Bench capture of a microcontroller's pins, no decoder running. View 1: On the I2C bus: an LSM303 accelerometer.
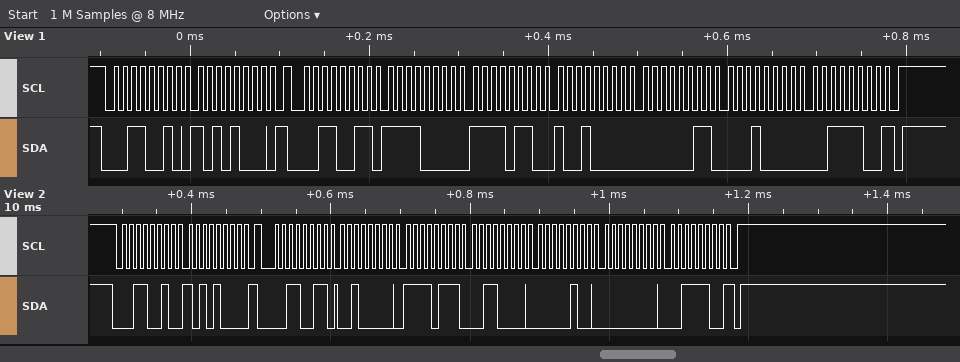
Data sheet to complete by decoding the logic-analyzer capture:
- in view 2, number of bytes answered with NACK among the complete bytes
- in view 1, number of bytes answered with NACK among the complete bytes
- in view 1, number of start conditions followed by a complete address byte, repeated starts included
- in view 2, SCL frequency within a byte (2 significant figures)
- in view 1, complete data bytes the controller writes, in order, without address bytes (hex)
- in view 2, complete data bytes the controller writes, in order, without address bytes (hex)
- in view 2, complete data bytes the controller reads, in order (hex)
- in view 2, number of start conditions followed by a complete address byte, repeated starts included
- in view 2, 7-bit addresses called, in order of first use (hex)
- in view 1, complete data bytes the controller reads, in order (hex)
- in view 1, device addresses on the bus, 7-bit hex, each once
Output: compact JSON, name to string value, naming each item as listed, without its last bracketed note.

{"in view 2, number of bytes answered with NACK among the complete bytes": "1", "in view 1, number of bytes answered with NACK among the complete bytes": "1", "in view 1, number of start conditions followed by a complete address byte, repeated starts included": "2", "in view 2, SCL frequency within a byte": "100 kHz", "in view 1, complete data bytes the controller writes, in order, without address bytes": "A8", "in view 2, complete data bytes the controller writes, in order, without address bytes": "A8", "in view 2, complete data bytes the controller reads, in order": "20 F7 30 04 00 3C", "in view 2, number of start conditions followed by a complete address byte, repeated starts included": "2", "in view 2, 7-bit addresses called, in order of first use": "0x19", "in view 1, complete data bytes the controller reads, in order": "F0 F6 90 03 10 3C", "in view 1, device addresses on the bus, 7-bit hex, each once": "0x19"}
